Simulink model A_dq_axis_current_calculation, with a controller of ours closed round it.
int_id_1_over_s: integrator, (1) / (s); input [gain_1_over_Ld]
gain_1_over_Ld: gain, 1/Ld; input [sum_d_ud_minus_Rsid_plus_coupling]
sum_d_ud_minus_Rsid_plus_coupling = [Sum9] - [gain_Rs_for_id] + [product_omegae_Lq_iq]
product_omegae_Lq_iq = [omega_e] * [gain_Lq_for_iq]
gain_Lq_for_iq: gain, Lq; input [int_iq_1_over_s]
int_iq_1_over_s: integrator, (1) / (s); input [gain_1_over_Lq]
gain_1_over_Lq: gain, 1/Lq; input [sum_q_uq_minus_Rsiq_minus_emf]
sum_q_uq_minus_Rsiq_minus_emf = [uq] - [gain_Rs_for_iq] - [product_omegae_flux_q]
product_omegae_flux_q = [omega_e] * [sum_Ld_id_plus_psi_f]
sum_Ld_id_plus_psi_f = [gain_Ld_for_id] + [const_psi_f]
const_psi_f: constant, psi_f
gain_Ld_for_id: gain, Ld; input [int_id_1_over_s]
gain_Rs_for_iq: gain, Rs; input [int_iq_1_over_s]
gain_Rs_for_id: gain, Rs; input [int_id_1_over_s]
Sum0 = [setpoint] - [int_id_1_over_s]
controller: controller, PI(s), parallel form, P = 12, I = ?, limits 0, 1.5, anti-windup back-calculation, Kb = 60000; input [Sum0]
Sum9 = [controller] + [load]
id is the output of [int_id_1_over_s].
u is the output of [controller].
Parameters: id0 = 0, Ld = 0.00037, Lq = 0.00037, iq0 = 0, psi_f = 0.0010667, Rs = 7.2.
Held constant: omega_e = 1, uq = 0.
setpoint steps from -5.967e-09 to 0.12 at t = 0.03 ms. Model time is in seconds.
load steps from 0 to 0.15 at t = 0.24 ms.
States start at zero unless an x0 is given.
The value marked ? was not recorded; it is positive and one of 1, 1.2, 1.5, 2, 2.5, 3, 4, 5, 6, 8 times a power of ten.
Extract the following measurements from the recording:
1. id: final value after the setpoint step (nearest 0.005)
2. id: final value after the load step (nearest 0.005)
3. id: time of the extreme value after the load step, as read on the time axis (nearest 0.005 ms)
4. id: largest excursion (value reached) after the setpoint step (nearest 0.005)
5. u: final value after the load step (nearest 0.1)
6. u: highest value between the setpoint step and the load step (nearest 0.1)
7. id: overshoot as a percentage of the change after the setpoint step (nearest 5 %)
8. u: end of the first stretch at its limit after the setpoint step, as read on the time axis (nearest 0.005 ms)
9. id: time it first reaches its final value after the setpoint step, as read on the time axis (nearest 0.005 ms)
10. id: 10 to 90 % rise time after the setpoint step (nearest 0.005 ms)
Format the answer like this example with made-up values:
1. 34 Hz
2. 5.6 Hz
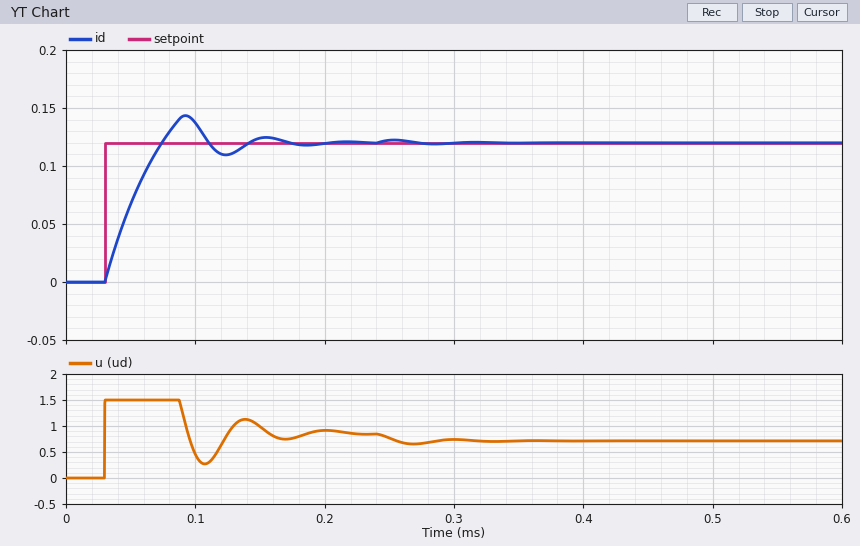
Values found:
1. 0.120
2. 0.120
3. 0.255 ms
4. 0.145
5. 0.7
6. 1.5
7. 20 %
8. 0.090 ms
9. 0.075 ms
10. 0.035 ms
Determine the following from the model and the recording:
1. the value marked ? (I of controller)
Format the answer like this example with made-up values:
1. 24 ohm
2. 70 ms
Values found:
1. 4e+06
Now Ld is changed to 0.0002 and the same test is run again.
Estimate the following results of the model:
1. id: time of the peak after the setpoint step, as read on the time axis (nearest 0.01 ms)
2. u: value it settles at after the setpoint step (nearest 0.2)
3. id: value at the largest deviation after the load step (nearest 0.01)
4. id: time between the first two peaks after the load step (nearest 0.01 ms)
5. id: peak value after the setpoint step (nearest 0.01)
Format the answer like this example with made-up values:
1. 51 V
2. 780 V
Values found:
1. 0.07 ms
2. 0.8
3. 0.12
4. 0.05 ms
5. 0.15
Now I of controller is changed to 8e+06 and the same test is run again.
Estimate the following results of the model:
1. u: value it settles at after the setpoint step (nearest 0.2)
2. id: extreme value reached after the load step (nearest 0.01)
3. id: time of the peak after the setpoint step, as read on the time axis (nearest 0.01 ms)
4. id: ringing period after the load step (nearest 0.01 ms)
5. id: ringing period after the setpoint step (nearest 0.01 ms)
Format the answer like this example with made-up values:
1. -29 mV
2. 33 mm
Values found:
1. 0.8
2. 0.12
3. 0.09 ms
4. 0.04 ms
5. 0.04 ms
